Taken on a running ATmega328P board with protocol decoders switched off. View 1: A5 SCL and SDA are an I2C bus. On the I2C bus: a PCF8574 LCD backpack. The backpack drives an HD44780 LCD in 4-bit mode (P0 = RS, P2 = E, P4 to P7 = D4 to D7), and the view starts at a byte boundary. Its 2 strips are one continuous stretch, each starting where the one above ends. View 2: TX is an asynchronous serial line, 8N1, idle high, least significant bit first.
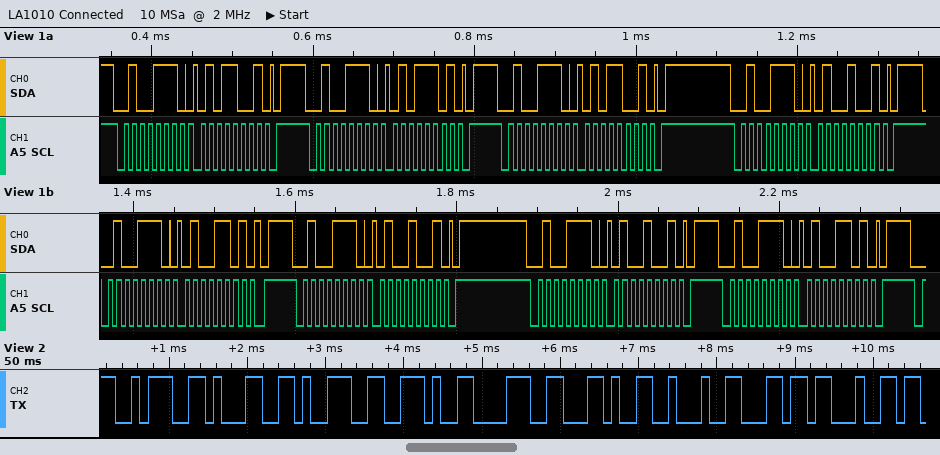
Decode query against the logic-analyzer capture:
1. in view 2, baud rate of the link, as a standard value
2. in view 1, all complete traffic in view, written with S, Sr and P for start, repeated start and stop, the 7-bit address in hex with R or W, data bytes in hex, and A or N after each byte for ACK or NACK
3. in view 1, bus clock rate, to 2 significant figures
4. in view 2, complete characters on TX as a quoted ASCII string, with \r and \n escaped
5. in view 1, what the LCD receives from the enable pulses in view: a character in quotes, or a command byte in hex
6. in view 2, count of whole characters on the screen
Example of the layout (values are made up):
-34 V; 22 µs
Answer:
9600 baud; S 27W A 59 A P S 27W A 5D A P S 27W A 59 A P S 27W A 49 A P S 27W A 4D A P S 27W A 49 A P S 27W A 49 A P S 27W A 4D A P; 100 kHz; ":19.8,\"ld"; 'T'; 9
